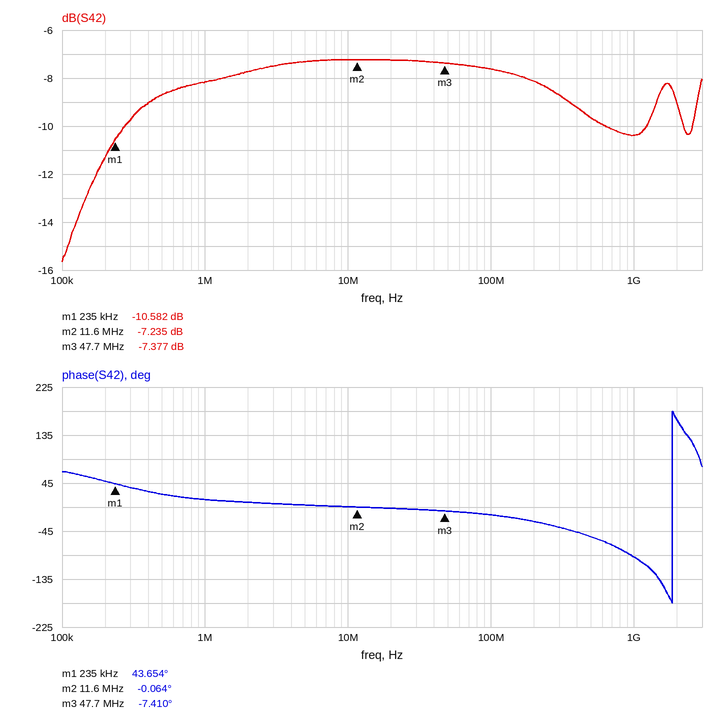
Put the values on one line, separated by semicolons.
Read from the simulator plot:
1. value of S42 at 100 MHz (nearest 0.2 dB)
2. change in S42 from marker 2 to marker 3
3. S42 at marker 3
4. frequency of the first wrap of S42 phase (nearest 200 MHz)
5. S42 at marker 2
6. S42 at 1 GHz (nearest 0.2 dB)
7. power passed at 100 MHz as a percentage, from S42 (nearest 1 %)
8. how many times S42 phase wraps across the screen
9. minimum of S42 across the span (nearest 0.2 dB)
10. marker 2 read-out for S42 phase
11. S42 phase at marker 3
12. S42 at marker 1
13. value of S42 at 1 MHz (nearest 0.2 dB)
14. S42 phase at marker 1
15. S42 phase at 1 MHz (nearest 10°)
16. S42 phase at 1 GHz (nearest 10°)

-7.6 dB; -0.142 dB; -7.377 dB; 1.8 GHz; -7.235 dB; -10.4 dB; 17 %; 1; -15.6 dB; -0.064°; -7.410°; -10.582 dB; -8.2 dB; 43.654°; 10°; -90°
